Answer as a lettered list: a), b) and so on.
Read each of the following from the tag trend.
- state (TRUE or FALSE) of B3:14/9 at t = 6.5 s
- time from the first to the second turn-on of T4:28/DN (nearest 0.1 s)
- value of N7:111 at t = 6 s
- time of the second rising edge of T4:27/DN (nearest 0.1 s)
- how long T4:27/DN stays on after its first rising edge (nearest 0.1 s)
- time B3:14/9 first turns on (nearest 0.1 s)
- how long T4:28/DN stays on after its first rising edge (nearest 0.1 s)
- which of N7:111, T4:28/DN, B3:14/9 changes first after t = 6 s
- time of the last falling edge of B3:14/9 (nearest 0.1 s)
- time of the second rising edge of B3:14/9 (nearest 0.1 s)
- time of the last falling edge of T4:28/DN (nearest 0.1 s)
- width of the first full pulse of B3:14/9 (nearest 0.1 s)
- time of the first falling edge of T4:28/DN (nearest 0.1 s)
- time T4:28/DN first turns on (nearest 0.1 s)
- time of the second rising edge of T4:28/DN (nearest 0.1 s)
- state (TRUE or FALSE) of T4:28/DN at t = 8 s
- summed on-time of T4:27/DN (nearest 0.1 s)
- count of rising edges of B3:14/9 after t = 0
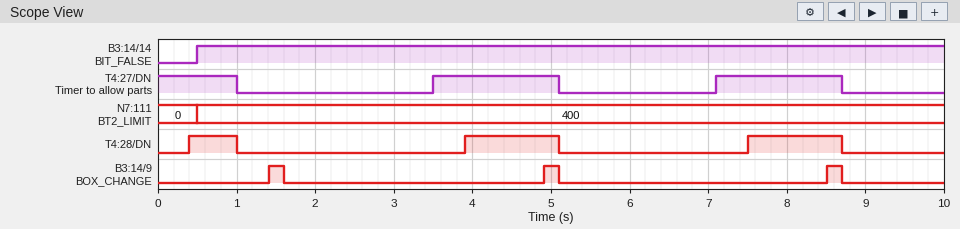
a) FALSE
b) 3.5 s
c) 400
d) 7.1 s
e) 1.6 s
f) 1.4 s
g) 0.6 s
h) T4:28/DN
i) 8.7 s
j) 4.9 s
k) 8.7 s
l) 0.2 s
m) 1.0 s
n) 0.4 s
o) 3.9 s
p) TRUE
q) 4.2 s
r) 3
